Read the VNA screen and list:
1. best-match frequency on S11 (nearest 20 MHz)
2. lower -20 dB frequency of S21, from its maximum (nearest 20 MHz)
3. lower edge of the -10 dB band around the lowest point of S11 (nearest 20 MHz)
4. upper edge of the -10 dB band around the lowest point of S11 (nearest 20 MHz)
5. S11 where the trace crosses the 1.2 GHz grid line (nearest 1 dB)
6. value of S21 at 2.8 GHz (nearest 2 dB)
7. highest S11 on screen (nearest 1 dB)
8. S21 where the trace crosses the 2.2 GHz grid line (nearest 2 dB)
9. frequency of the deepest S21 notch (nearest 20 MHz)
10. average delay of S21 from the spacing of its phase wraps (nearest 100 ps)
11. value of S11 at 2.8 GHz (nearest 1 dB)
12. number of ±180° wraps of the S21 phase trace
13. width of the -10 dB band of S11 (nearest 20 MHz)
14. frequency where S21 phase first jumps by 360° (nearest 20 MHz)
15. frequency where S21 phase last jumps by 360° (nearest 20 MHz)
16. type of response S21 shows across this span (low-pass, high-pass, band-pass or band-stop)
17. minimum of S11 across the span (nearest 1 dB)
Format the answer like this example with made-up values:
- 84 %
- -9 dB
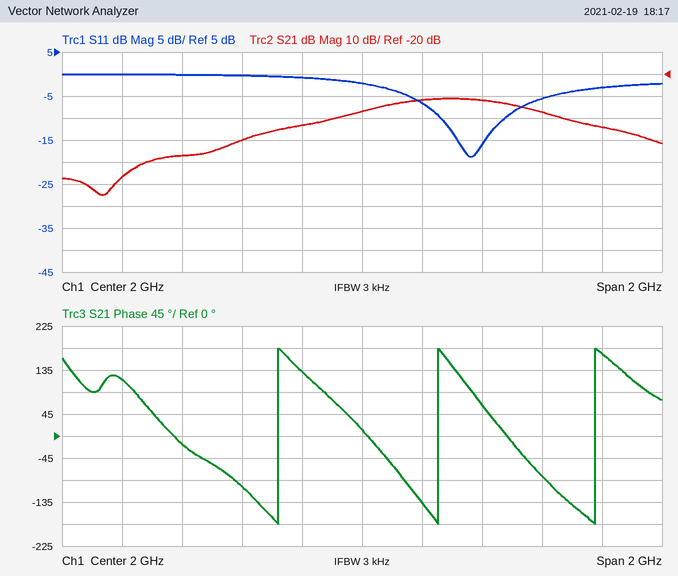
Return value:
- 2.36 GHz
- 1.58 GHz
- 2.26 GHz
- 2.48 GHz
- 0 dB
- -44 dB
- 0 dB
- -32 dB
- 1.14 GHz
- 1.9 ns
- -3 dB
- 3
- 220 MHz
- 1.72 GHz
- 2.78 GHz
- band-pass
- -19 dB
